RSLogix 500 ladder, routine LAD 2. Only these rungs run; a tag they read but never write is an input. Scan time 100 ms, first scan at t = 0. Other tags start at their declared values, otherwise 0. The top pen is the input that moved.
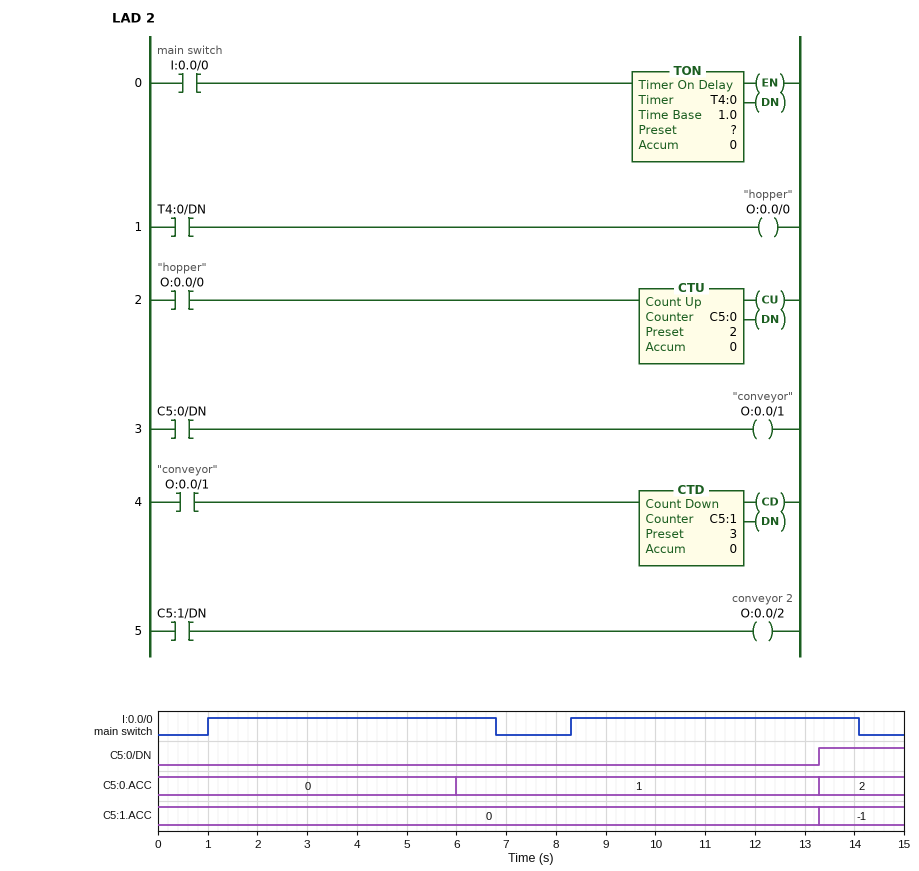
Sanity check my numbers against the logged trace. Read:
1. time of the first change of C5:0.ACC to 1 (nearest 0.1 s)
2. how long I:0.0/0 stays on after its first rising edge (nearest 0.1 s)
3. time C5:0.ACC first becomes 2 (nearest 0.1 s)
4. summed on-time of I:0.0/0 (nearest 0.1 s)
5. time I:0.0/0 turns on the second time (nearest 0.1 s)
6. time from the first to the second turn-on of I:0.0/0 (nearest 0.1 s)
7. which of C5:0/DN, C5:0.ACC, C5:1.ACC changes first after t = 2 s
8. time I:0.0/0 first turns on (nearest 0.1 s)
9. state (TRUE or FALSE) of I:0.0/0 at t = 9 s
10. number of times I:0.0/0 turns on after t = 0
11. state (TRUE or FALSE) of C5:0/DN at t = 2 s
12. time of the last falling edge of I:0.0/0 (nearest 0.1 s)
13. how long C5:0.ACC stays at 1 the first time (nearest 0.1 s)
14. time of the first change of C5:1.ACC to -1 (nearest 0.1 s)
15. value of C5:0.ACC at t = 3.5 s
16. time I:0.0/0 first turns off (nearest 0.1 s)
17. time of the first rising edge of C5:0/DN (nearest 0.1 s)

6.0 s
5.8 s
13.3 s
11.6 s
8.3 s
7.3 s
C5:0.ACC
1.0 s
TRUE
2
FALSE
14.1 s
7.3 s
13.3 s
0
6.8 s
13.3 s
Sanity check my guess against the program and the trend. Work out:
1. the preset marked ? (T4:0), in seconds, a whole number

5 s
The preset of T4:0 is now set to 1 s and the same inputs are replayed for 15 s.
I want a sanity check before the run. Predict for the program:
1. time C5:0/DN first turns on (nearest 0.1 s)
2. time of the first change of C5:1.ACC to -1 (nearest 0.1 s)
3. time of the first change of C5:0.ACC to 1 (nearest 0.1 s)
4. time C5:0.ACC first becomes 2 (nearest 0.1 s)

9.3 s
9.3 s
2.0 s
9.3 s
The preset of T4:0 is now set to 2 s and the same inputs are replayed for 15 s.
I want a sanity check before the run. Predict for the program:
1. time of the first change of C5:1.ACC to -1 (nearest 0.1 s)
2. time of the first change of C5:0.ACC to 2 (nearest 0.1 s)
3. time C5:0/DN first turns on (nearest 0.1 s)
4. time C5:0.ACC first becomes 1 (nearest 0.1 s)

10.3 s
10.3 s
10.3 s
3.0 s
